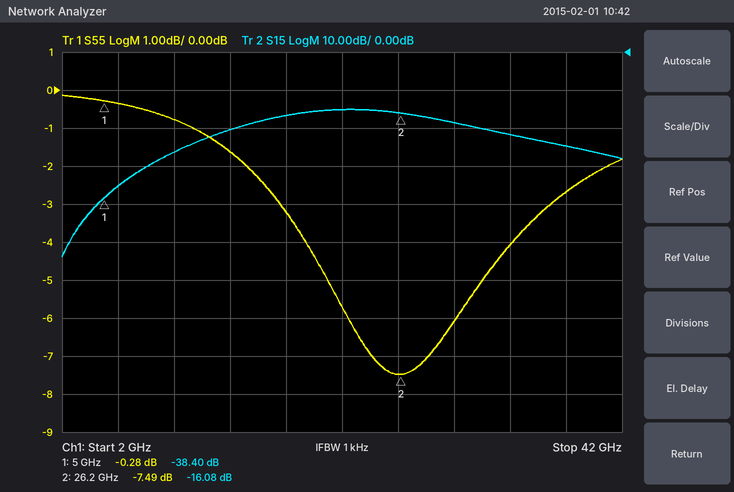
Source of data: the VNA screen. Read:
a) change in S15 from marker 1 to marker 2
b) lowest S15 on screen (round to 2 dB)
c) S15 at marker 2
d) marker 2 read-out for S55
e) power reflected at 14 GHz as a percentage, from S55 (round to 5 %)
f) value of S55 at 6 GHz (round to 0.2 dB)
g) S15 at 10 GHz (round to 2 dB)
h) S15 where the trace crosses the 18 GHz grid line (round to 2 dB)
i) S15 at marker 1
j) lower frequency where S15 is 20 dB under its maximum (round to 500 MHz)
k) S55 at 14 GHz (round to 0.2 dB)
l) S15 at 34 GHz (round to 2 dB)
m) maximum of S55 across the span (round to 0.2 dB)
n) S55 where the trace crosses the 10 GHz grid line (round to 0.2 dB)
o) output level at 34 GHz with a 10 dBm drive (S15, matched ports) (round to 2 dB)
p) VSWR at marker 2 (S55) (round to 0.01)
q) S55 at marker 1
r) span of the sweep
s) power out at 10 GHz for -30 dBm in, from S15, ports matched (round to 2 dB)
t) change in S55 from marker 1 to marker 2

22.32 dB
-54 dB
-16.08 dB
-7.49 dB
70 %
-0.4 dB
-26 dB
-16 dB
-38.40 dB
6.0 GHz
-1.6 dB
-22 dB
-0.2 dB
-0.8 dB
-12 dBm
2.46
-0.28 dB
40 GHz
-56 dBm
-7.21 dB
